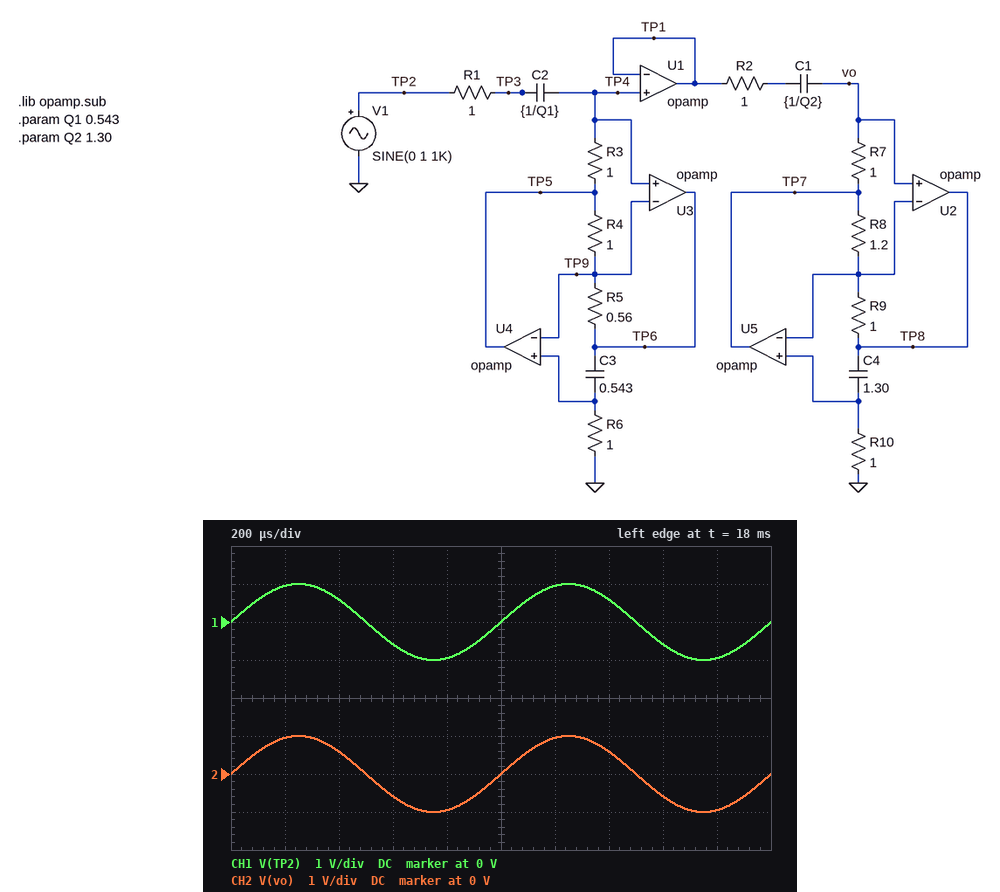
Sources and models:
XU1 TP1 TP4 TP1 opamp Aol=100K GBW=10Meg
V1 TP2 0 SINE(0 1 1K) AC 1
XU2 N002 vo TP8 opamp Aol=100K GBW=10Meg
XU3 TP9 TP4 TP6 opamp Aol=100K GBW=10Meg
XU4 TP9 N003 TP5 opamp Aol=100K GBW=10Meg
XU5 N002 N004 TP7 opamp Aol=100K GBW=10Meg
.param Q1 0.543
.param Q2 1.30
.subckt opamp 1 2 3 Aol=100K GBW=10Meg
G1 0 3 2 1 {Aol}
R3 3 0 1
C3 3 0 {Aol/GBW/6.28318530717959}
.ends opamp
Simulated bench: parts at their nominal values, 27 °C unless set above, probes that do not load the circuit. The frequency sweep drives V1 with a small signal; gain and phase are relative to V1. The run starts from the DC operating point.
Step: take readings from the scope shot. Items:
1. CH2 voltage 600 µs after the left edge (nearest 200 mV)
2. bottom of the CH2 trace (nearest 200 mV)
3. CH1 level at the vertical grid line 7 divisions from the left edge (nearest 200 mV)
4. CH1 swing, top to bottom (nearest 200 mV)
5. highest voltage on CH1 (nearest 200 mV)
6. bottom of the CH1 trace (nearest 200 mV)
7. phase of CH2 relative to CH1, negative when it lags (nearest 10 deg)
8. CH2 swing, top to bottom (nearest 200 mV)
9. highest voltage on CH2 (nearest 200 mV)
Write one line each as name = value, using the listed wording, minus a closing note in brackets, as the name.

CH2 voltage 600 µs after the left edge = -600 mV
bottom of the CH2 trace = -1.0 V
CH1 level at the vertical grid line 7 divisions from the left edge = 600 mV
CH1 swing, top to bottom = 2.0 V
highest voltage on CH1 = 1.0 V
bottom of the CH1 trace = -1.0 V
phase of CH2 relative to CH1, negative when it lags = 0 deg
CH2 swing, top to bottom = 2.0 V
highest voltage on CH2 = 1.0 V
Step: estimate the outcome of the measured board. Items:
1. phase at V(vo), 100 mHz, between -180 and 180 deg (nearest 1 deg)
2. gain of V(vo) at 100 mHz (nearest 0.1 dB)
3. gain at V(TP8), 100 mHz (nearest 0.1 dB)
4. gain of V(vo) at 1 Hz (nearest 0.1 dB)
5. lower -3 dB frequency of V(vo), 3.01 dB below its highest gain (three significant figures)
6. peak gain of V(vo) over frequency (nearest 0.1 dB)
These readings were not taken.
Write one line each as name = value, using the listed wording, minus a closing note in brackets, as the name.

phase at V(vo), 100 mHz, between -180 and 180 deg = -92 deg
gain of V(vo) at 100 mHz = -24.0 dB
gain at V(TP8), 100 mHz = -20.0 dB
gain of V(vo) at 1 Hz = -0.6 dB
lower -3 dB frequency of V(vo), 3.01 dB below its highest gain = 340 mHz
peak gain of V(vo) over frequency = 0 dB
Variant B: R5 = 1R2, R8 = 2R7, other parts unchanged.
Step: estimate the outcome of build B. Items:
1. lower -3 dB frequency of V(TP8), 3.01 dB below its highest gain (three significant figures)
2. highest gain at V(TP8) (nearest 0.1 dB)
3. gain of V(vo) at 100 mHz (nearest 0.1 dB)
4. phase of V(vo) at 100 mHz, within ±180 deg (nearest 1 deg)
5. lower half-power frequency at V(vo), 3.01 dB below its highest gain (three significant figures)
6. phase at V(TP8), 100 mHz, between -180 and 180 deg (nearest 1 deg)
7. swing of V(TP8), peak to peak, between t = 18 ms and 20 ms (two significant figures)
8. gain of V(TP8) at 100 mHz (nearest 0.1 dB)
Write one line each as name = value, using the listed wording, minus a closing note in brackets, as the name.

lower -3 dB frequency of V(TP8), 3.01 dB below its highest gain = 252 mHz
highest gain at V(TP8) = 0.1 dB
gain of V(vo) at 100 mHz = -25.1 dB
phase of V(vo) at 100 mHz, within ±180 deg = -95 deg
lower half-power frequency at V(vo), 3.01 dB below its highest gain = 270 mHz
phase at V(TP8), 100 mHz, between -180 and 180 deg = -146 deg
swing of V(TP8), peak to peak, between t = 18 ms and 20 ms = 2.0 V
gain of V(TP8) at 100 mHz = -21.1 dB
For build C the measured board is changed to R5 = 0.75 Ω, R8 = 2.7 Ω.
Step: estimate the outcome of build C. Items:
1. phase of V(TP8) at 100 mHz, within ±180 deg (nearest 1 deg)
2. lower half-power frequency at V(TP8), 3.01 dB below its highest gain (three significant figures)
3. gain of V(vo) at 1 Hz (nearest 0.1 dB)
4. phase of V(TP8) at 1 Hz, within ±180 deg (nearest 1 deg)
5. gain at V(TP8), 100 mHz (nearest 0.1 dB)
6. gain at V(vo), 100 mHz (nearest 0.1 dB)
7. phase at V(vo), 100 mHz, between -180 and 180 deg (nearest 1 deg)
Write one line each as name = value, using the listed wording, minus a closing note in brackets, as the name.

phase of V(TP8) at 100 mHz, within ±180 deg = -139 deg
lower half-power frequency at V(TP8), 3.01 dB below its highest gain = 319 mHz
gain of V(vo) at 1 Hz = -0.3 dB
phase of V(TP8) at 1 Hz, within ±180 deg = 35 deg
gain at V(TP8), 100 mHz = -25.8 dB
gain at V(vo), 100 mHz = -29.7 dB
phase at V(vo), 100 mHz, between -180 and 180 deg = -88 deg
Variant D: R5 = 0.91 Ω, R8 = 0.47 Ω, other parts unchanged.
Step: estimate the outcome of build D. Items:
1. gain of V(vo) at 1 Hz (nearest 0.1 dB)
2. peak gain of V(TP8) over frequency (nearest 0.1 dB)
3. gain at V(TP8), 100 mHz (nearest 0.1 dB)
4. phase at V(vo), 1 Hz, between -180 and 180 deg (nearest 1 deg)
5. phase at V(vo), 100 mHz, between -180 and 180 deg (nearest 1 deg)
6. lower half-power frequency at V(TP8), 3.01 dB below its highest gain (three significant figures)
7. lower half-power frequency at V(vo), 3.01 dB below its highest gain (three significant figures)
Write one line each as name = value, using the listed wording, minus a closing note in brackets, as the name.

gain of V(vo) at 1 Hz = -0.1 dB
peak gain of V(TP8) over frequency = 0.1 dB
gain at V(TP8), 100 mHz = -3.0 dB
phase at V(vo), 1 Hz, between -180 and 180 deg = 22 deg
phase at V(vo), 100 mHz, between -180 and 180 deg = -133 deg
lower half-power frequency at V(TP8), 3.01 dB below its highest gain = 100 mHz
lower half-power frequency at V(vo), 3.01 dB below its highest gain = 123 mHz
